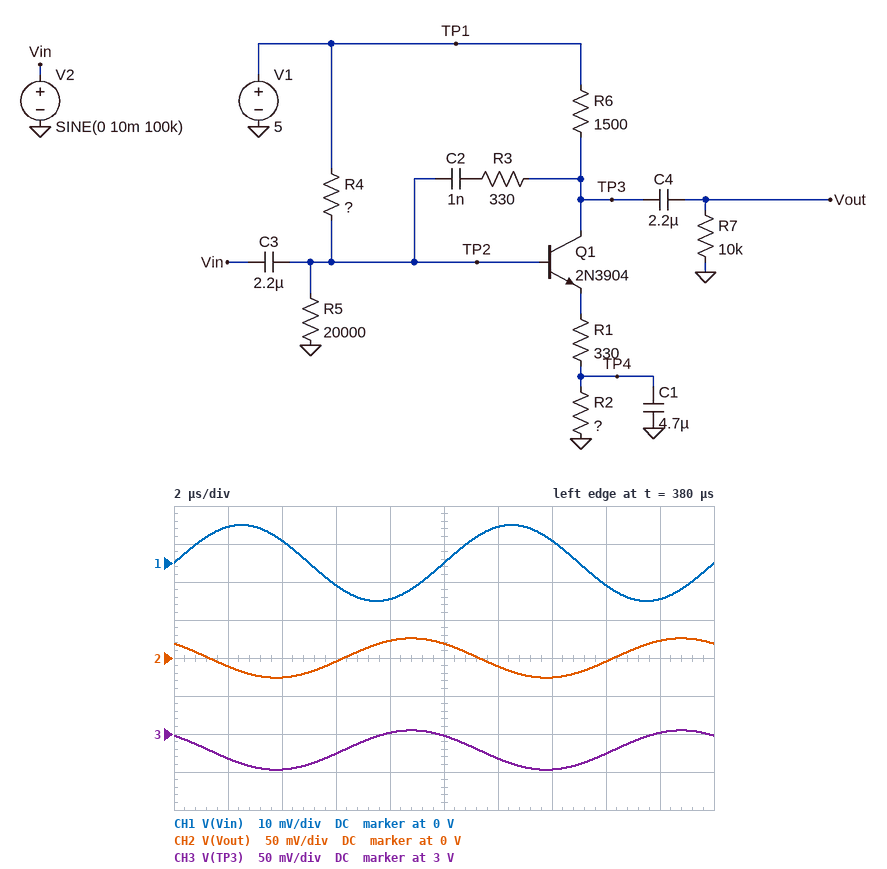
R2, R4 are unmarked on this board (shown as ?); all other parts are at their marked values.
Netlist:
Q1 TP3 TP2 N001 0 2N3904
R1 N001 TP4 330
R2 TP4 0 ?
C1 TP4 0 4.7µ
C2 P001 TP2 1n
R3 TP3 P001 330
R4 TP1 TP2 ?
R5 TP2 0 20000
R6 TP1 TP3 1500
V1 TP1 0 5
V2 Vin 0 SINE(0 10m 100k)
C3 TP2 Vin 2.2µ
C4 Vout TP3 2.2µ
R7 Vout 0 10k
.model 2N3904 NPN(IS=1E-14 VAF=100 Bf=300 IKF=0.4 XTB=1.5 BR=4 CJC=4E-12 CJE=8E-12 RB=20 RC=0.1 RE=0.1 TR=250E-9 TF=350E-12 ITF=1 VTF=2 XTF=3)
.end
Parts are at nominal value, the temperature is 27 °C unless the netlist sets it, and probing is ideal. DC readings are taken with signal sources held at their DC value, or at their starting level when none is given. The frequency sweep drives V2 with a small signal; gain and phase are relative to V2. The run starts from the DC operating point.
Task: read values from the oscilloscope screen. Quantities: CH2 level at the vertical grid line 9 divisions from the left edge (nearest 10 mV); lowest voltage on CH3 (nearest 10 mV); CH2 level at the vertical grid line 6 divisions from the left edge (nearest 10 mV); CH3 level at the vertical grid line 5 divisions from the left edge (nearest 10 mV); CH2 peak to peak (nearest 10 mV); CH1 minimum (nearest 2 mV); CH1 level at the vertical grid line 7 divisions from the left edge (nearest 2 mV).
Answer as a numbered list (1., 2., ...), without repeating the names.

1. 20 mV
2. 2.95 V
3. -10 mV
4. 3.00 V
5. 50 mV
6. -10 mV
7. 6 mV
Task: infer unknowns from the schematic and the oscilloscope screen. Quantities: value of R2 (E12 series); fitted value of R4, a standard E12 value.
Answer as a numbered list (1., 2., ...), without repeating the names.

1. 390 Ω
2. 39 kΩ
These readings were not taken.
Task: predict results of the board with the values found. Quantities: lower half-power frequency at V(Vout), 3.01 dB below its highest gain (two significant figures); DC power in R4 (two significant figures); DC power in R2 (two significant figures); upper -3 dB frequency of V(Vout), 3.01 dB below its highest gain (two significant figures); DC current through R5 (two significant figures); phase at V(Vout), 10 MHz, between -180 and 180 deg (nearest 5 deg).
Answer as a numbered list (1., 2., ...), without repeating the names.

1. 140 Hz
2. 290 µW
3. 710 µW
4. 98 kHz
5. 82 µA
6. 65 deg
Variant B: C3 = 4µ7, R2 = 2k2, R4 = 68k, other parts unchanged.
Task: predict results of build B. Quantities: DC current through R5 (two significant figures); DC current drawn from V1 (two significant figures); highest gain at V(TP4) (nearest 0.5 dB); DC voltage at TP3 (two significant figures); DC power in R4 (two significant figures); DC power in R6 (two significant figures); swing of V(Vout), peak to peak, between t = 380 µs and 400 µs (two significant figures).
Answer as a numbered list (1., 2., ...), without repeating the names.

1. 56 µA
2. 260 µA
3. -2.0 dB
4. 4.7 V
5. 220 µW
6. 61 µW
7. 40 mV
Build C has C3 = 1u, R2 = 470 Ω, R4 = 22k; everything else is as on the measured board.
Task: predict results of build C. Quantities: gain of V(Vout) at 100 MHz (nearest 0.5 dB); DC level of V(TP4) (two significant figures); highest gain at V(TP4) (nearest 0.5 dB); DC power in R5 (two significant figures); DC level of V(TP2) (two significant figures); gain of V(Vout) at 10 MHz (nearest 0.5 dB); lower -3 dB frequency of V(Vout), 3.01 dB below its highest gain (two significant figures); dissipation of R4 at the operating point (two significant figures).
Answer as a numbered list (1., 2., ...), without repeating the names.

1. -2.0 dB
2. 960 mV
3. -5.5 dB
4. 270 µW
5. 2.3 V
6. -16.0 dB
7. 140 Hz
8. 330 µW
